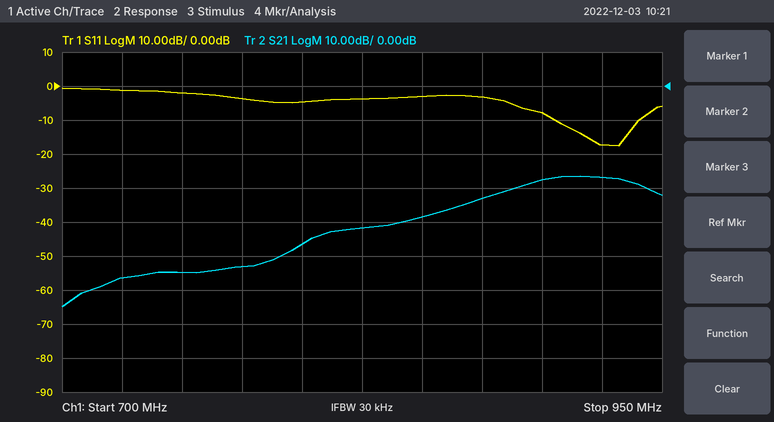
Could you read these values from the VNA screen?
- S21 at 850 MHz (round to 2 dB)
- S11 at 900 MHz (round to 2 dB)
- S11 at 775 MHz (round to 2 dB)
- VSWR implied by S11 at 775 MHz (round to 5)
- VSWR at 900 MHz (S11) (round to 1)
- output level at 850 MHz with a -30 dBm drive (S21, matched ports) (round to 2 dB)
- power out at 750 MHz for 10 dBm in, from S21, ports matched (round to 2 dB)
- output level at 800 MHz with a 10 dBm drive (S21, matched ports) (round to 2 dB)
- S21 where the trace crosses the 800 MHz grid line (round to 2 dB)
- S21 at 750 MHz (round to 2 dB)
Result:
-38 dB
-8 dB
-4 dB
5
2
-68 dBm
-44 dBm
-36 dBm
-46 dB
-54 dB
